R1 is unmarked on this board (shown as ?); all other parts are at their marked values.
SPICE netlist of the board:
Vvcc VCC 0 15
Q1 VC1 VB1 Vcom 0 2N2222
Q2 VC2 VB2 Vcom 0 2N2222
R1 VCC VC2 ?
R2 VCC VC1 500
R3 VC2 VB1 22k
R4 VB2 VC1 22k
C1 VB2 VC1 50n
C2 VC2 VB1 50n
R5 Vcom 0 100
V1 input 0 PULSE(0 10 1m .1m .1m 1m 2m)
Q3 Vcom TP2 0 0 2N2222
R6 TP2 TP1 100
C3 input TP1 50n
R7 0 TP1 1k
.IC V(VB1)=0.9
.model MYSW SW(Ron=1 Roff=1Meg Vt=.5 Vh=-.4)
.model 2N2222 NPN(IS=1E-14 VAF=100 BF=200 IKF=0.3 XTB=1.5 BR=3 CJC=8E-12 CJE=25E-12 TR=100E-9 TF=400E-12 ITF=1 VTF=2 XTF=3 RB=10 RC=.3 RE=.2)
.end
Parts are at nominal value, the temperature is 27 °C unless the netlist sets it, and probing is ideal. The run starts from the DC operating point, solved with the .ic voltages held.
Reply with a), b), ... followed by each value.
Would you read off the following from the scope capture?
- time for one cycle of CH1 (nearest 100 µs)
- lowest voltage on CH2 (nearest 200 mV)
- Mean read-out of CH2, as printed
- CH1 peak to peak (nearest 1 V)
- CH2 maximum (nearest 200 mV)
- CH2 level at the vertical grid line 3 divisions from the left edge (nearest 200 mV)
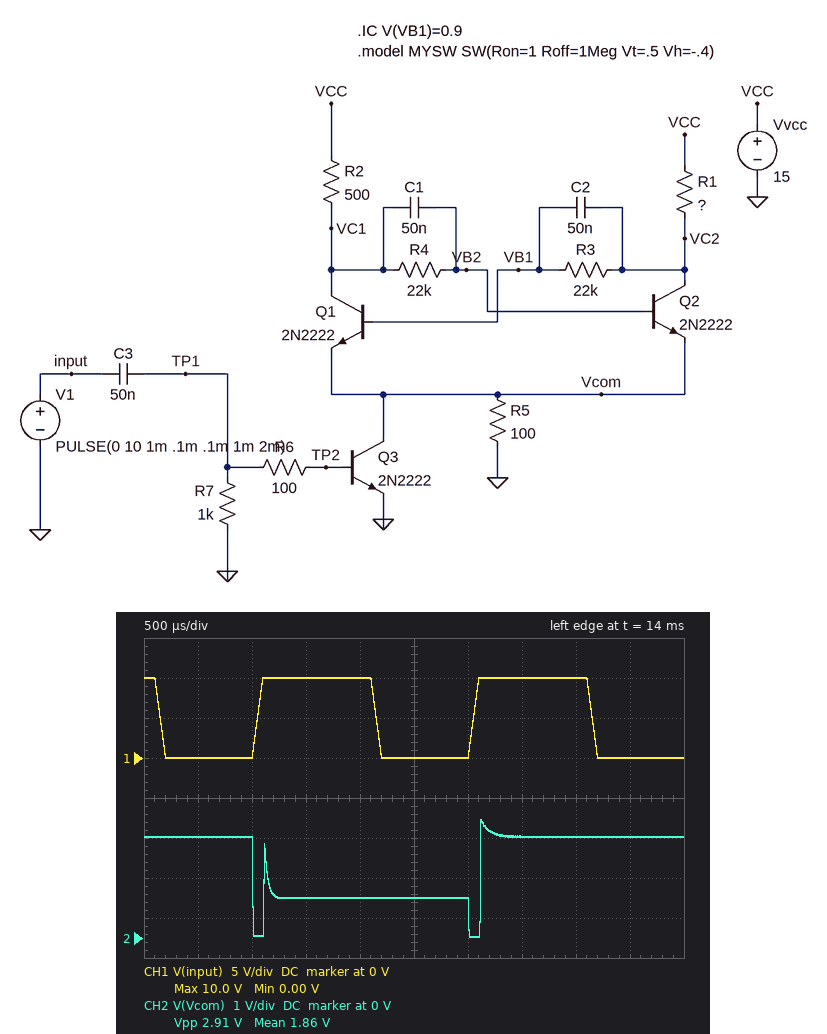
a) 2.0 ms
b) 0 V
c) 1.86 V
d) 10 V
e) 3.0 V
f) 1.0 V
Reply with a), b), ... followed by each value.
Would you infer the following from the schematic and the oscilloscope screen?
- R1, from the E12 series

a) 1.5 kΩ
